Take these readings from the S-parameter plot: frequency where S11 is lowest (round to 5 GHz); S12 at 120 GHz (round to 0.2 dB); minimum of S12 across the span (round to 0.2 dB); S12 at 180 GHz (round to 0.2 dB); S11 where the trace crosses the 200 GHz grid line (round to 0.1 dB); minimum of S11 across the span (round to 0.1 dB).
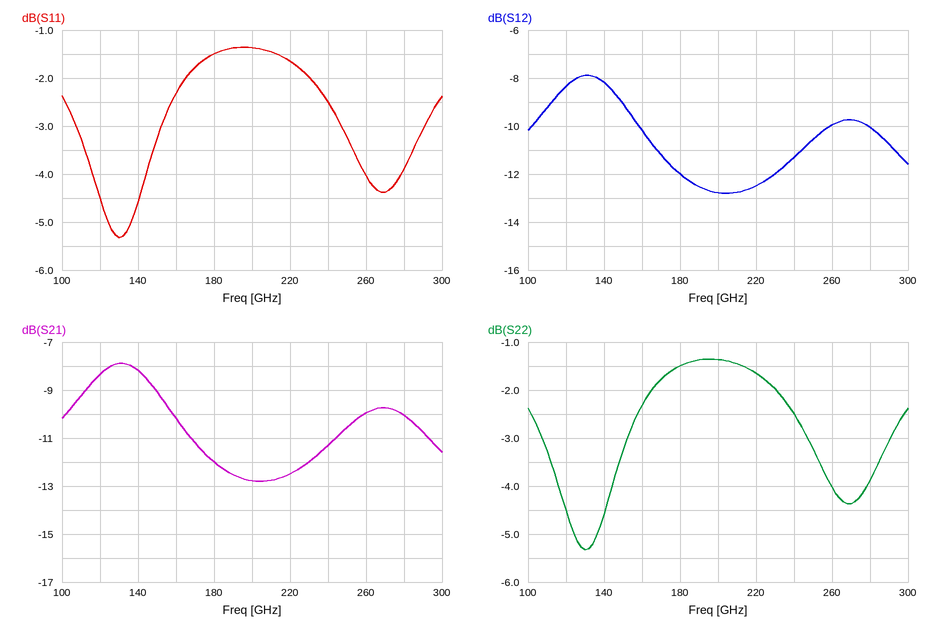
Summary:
130 GHz
-8.4 dB
-12.8 dB
-12.0 dB
-1.4 dB
-5.3 dB
